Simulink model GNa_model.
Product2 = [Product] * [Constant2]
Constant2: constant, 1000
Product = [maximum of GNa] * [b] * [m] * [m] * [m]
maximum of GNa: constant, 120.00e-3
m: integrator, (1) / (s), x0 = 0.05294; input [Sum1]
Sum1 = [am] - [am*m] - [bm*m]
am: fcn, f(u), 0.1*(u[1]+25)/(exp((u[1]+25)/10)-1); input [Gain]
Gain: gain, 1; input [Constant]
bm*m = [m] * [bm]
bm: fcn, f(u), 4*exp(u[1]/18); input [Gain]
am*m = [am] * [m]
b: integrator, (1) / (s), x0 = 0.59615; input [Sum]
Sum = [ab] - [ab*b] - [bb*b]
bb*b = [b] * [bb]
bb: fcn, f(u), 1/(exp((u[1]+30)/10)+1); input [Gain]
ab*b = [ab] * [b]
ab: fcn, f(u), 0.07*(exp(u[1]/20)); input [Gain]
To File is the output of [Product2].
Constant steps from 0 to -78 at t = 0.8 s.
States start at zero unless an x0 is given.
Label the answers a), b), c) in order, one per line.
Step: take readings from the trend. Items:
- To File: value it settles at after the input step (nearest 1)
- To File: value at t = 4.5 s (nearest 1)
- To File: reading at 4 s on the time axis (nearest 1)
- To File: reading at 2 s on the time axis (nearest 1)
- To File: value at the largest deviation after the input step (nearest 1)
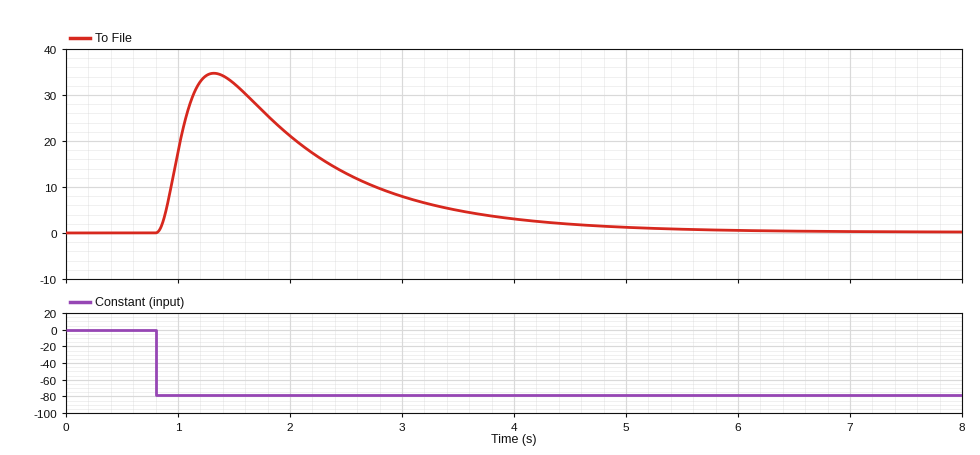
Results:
a) 0
b) 2
c) 3
d) 21
e) 35
